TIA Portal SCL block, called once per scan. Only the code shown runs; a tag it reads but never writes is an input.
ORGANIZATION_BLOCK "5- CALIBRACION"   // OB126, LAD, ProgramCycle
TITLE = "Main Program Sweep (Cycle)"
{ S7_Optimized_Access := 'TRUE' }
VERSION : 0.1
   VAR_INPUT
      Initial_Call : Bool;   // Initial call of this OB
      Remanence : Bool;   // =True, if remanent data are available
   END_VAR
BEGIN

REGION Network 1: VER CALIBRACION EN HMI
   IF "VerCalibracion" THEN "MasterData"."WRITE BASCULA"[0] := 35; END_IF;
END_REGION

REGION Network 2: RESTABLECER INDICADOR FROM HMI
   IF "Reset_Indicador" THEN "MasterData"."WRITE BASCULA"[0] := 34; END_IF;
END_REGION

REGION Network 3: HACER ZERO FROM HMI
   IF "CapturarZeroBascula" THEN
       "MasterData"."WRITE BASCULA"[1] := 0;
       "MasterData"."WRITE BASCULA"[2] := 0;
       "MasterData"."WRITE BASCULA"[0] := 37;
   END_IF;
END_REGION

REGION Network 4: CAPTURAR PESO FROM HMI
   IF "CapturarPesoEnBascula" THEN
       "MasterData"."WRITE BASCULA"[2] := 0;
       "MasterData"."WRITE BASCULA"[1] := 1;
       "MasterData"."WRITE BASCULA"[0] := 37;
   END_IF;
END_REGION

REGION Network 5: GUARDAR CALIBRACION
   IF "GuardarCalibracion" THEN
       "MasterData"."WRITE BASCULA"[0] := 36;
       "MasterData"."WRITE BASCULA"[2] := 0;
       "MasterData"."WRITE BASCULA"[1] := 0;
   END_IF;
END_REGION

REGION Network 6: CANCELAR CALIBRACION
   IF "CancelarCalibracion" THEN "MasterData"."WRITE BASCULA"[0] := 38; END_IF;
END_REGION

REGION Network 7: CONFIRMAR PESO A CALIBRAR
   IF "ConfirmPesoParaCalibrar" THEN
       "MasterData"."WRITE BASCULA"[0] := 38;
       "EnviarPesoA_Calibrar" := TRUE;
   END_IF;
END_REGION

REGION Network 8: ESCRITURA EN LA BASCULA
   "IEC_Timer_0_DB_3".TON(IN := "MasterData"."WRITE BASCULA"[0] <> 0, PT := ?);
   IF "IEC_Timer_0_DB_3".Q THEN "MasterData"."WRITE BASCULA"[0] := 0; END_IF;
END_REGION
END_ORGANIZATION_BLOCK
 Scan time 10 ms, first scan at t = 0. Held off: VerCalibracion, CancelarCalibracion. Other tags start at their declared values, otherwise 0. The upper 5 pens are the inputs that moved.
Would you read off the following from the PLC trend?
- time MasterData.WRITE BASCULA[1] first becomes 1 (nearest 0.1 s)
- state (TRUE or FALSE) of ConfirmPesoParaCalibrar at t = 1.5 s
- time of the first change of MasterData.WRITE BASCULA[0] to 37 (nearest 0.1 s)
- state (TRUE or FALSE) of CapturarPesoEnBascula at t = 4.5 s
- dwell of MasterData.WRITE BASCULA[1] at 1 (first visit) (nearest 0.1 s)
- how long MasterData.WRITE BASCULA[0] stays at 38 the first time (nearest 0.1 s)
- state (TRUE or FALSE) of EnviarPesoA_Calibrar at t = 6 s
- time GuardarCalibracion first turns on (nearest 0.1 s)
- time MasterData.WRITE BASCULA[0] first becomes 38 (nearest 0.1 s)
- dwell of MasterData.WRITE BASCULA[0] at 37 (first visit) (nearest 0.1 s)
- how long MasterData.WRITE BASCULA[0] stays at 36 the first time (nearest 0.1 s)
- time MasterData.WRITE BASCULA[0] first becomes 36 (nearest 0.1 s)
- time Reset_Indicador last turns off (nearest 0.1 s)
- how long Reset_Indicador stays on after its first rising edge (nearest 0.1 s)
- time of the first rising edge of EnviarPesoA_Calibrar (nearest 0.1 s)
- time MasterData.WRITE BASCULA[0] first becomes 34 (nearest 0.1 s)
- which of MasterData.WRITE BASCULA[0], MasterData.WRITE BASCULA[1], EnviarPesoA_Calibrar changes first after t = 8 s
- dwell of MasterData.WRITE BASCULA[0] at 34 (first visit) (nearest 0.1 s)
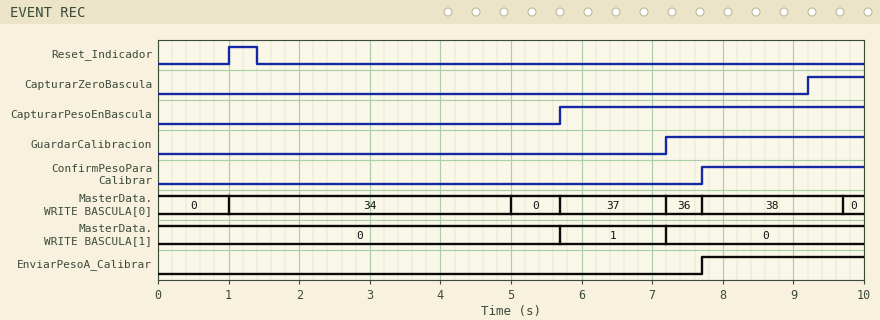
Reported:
5.7 s
FALSE
5.7 s
FALSE
1.5 s
2.0 s
FALSE
7.2 s
7.7 s
1.5 s
0.5 s
7.2 s
1.4 s
0.4 s
7.7 s
1.0 s
MasterData.WRITE BASCULA[0]
4.0 s
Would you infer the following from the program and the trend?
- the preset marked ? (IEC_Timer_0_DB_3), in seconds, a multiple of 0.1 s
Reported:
4.0 s
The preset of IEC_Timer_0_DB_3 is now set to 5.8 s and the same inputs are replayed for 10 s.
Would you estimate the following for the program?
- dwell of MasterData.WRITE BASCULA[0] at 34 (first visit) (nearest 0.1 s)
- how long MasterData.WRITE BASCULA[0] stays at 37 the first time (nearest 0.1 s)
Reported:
4.7 s
1.1 s
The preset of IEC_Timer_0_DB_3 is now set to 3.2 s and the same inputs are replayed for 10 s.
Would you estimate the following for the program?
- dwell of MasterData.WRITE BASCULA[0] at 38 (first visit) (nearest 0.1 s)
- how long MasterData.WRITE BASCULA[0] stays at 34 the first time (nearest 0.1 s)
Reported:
1.2 s
3.2 s
